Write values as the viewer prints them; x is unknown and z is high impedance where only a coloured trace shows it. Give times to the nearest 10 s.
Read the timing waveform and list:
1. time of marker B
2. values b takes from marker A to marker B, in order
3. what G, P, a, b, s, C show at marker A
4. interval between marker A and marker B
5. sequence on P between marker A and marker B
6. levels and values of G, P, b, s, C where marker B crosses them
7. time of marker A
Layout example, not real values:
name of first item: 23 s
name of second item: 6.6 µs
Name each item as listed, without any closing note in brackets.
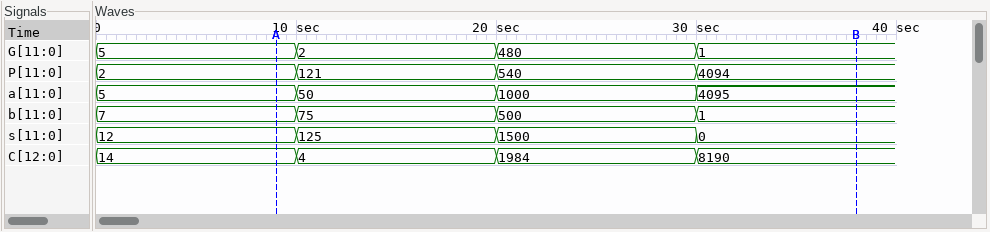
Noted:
time of marker B: 40 s
values b takes from marker A to marker B, in order: 7, 75, 500, 1
what G, P, a, b, s, C show at marker A: G=5, P=2, a=5, b=7, s=12, C=14
interval between marker A and marker B: 30 s
sequence on P between marker A and marker B: 2, 121, 540, 4094
levels and values of G, P, b, s, C where marker B crosses them: G=1, P=4094, b=1, s=0, C=8190
time of marker A: 10 s
